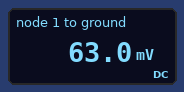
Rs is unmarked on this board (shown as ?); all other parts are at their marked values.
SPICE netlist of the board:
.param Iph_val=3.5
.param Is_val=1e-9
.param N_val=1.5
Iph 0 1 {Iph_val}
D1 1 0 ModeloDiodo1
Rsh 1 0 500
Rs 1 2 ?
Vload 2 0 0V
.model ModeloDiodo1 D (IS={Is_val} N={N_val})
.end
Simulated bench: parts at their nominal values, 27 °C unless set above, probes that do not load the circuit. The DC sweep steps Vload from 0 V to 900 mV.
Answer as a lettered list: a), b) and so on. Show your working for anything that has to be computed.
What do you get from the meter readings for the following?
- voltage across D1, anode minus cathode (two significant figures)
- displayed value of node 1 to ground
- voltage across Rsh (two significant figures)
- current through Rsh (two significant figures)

a) 63 mV = 63 mV
b) 63.0 mV
c) 63 mV = 63 mV
d) (63 mV) / 500 Ω = 130 µA
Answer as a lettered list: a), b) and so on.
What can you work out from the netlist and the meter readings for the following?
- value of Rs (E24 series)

a) 0.018 Ω
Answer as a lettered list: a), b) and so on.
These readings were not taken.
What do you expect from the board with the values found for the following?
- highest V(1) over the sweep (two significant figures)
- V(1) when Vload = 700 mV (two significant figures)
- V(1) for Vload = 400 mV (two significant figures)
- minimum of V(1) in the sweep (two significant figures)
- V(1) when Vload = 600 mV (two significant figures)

a) 870 mV
b) 760 mV
c) 460 mV
d) 63 mV
e) 660 mV
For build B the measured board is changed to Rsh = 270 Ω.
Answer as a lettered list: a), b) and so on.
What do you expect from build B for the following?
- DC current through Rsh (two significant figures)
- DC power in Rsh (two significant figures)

a) 230 µA
b) 15 µW
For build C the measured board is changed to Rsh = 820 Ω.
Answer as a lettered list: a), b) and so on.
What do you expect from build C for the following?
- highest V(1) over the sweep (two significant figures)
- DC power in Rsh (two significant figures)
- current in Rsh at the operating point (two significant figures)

a) 870 mV
b) 4.8 µW
c) 77 µA
